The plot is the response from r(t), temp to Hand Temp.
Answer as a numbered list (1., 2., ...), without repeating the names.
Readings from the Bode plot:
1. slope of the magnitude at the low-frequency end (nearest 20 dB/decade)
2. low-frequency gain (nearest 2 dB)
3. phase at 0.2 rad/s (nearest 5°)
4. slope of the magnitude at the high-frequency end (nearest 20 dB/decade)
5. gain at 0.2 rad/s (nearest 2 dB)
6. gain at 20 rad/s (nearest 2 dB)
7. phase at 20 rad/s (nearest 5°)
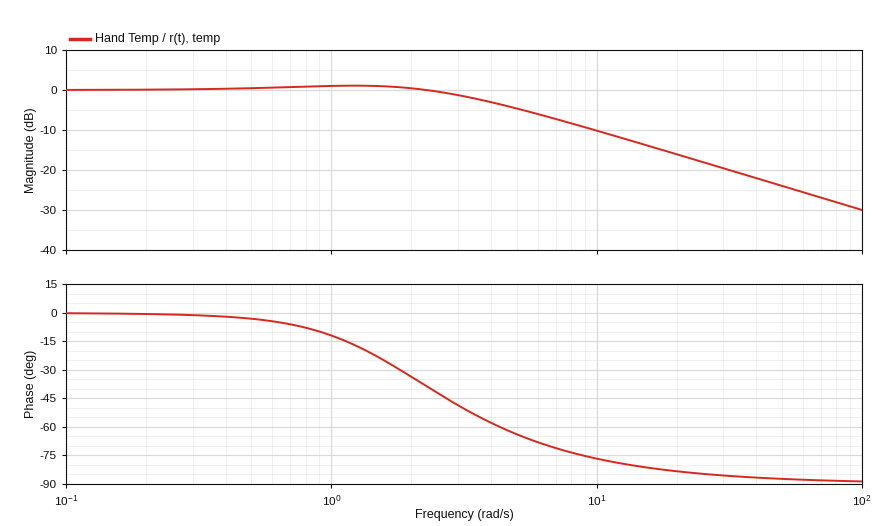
1. 0 dB/decade
2. 0 dB
3. 0°
4. -20 dB/decade
5. 0 dB
6. -16 dB
7. -85°
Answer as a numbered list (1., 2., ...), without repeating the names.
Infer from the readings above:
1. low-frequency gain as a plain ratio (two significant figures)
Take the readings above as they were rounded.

1. 1.0
